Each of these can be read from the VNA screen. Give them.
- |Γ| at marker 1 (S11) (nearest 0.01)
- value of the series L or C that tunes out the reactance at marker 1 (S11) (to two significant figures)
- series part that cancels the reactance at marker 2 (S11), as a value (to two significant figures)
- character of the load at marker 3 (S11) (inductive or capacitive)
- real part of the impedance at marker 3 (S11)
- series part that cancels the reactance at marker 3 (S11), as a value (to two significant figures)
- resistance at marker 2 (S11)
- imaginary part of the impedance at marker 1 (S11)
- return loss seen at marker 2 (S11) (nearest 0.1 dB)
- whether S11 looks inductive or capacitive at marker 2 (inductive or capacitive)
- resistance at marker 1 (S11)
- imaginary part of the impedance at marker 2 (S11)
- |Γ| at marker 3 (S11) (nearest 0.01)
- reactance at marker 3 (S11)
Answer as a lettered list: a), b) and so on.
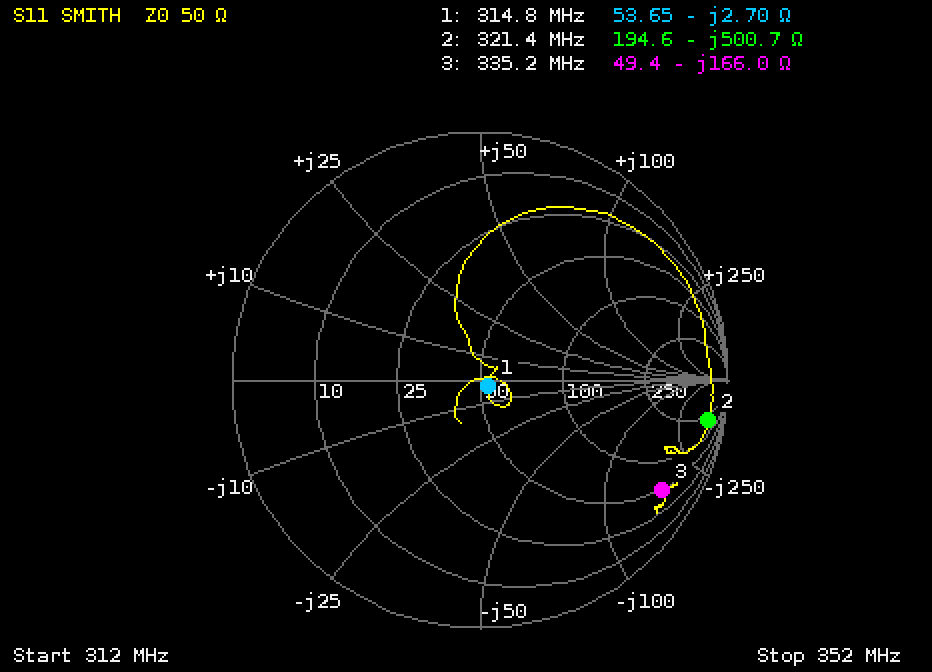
a) 0.04
b) 1.4 nH
c) 250 nH
d) capacitive
e) 49.4 Ω
f) 79 nH
g) 194.6 Ω
h) -2.70 Ω
i) 0.6 dB
j) capacitive
k) 53.65 Ω
l) -500.7 Ω
m) 0.86
n) -166.0 Ω
